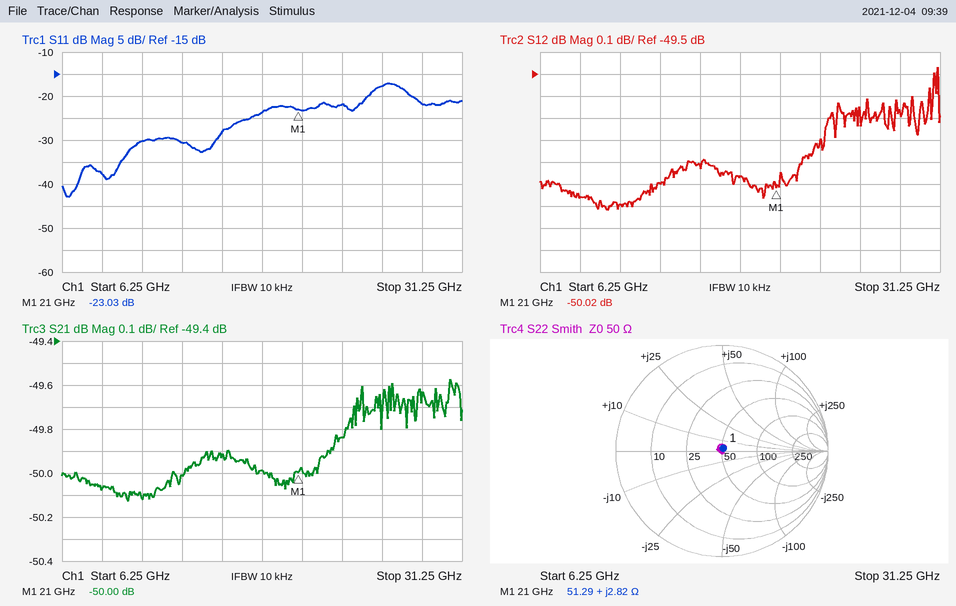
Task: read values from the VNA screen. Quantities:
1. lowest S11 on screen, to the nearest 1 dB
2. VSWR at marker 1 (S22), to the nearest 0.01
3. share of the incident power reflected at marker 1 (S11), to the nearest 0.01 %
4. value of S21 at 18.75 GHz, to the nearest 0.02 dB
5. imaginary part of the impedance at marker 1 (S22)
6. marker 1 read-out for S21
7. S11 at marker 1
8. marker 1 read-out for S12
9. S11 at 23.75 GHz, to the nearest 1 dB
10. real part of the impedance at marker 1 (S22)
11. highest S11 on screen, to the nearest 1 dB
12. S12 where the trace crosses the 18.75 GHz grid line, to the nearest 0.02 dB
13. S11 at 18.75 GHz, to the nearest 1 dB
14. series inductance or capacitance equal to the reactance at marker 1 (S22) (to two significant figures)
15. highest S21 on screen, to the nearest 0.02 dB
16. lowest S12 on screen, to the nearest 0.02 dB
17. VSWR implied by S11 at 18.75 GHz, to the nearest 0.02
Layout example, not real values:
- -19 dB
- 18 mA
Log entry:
- -43 dB
- 1.06
- 0.50 %
- -49.98 dB
- +2.82 Ω
- -50.00 dB
- -23.03 dB
- -50.02 dB
- -22 dB
- 51.29 Ω
- -17 dB
- -49.96 dB
- -24 dB
- 21 pH
- -49.58 dB
- -50.12 dB
- 1.14
